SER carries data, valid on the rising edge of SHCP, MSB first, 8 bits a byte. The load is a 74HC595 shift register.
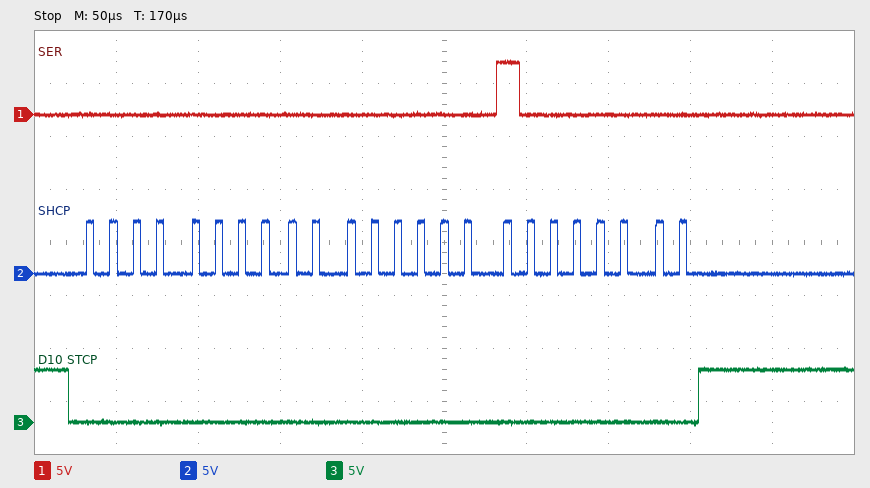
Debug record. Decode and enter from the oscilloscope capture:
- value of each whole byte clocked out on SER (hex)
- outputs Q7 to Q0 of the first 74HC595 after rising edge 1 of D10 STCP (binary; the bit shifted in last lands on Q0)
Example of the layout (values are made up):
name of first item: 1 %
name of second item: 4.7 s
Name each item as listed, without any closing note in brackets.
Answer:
value of each whole byte clocked out on SER: 00 00 80
outputs Q7 to Q0 of the first 74HC595 after rising edge 1 of D10 STCP: 10000000
